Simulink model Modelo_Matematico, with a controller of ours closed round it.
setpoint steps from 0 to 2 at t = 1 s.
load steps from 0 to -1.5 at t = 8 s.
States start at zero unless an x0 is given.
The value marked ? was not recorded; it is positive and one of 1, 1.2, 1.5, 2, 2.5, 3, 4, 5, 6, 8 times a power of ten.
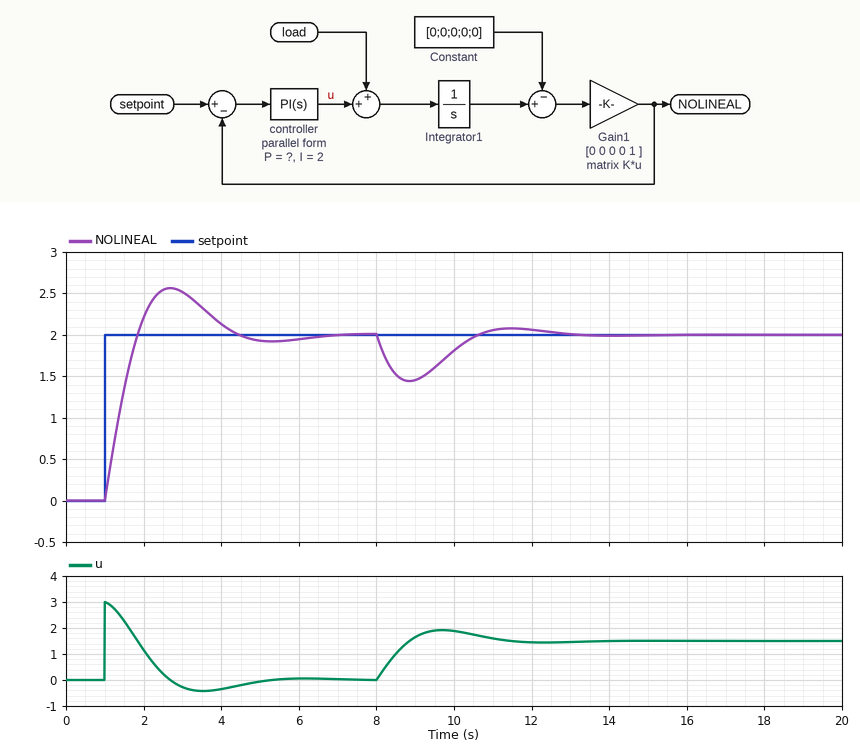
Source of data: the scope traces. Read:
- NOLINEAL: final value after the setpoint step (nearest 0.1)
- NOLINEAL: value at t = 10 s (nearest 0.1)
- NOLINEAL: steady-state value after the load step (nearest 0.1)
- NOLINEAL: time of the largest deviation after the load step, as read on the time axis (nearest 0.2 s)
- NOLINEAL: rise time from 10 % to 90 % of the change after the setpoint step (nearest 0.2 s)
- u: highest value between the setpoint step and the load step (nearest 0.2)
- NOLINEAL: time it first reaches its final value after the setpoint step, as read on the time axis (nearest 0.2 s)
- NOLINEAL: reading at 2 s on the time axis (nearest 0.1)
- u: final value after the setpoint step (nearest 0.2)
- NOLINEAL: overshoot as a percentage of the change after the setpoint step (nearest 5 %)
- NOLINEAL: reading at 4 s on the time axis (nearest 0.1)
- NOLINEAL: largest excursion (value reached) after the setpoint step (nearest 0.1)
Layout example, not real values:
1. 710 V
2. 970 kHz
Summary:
1. 2.0
2. 1.8
3. 2.0
4. 8.8 s
5. 0.6 s
6. 3.0
7. 1.8 s
8. 2.2
9. 0.0
10. 30 %
11. 2.1
12. 2.6
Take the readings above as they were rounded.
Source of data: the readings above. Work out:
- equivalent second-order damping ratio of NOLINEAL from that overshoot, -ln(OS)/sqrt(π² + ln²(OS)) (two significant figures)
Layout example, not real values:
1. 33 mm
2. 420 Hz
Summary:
1. 0.36
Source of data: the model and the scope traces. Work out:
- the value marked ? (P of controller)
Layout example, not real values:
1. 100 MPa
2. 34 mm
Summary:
1. 1.5
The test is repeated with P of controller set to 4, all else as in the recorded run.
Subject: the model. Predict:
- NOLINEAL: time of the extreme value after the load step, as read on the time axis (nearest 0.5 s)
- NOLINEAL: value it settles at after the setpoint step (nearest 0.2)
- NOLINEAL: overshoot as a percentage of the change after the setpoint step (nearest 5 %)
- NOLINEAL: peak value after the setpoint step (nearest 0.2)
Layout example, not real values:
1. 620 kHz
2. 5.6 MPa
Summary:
1. 8.5 s
2. 2.0
3. 10 %
4. 2.2
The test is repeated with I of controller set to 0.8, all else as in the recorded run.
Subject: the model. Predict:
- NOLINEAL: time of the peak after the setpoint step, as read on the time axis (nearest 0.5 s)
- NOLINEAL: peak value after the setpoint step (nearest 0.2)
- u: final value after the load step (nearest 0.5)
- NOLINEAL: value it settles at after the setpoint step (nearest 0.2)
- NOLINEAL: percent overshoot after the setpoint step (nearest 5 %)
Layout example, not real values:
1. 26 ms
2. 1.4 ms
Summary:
1. 3.5 s
2. 2.4
3. 1.5
4. 2.0
5. 15 %
